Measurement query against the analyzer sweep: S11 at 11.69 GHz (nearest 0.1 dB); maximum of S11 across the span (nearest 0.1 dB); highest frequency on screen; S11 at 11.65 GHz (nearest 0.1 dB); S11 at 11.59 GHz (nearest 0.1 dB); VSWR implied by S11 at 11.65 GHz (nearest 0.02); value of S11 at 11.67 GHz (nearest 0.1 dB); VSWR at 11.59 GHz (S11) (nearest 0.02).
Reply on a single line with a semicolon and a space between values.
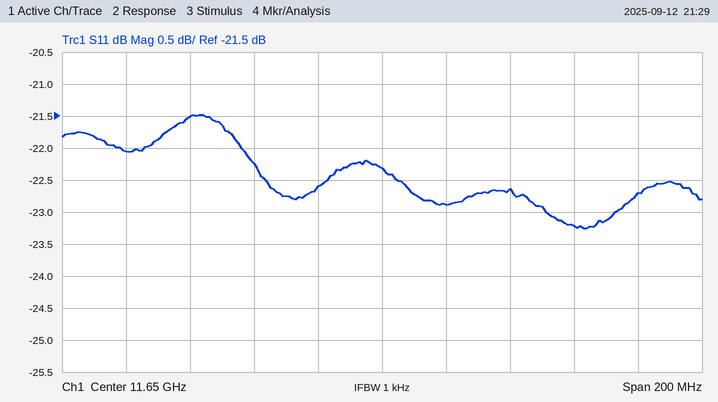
-22.6 dB; -21.5 dB; 11.75 GHz; -22.3 dB; -21.5 dB; 1.16; -22.9 dB; 1.18
